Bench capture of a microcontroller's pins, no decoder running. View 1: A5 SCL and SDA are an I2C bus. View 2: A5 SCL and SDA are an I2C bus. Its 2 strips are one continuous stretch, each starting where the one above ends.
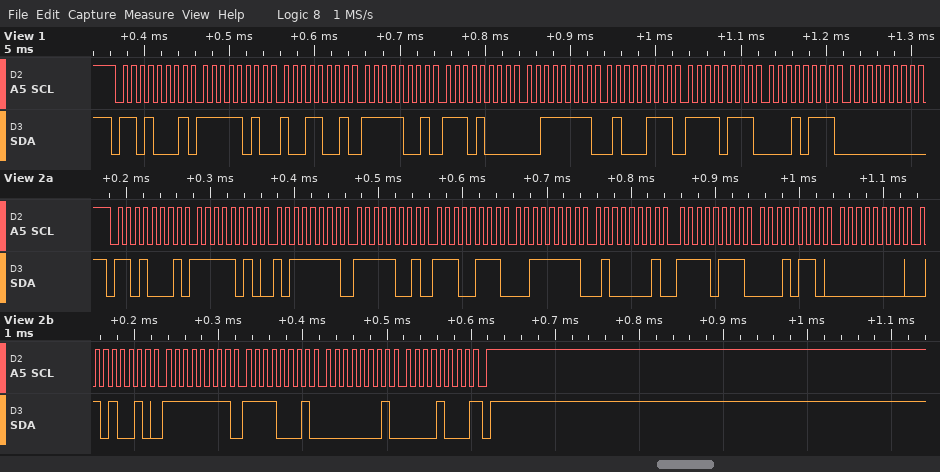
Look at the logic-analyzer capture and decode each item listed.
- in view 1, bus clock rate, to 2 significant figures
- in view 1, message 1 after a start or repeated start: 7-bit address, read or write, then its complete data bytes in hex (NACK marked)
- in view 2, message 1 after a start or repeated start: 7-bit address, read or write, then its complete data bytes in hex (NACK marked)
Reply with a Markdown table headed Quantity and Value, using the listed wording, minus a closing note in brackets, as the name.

| Quantity | Value |
|---|---|
| in view 1, bus clock rate, to 2 significant figures | 100 kHz |
| in view 1, message 1 after a start or repeated start: 7-bit address, read or write, then its complete data bytes in hex | 0x68 read: FA 99 F9 E8 3F 47 F7 17 00 |
| in view 2, message 1 after a start or repeated start: 7-bit address, read or write, then its complete data bytes in hex | 0x68 read: FA BF F9 E7 3F 41 F7 16 00 52 FF F1 01 08 NACK |
